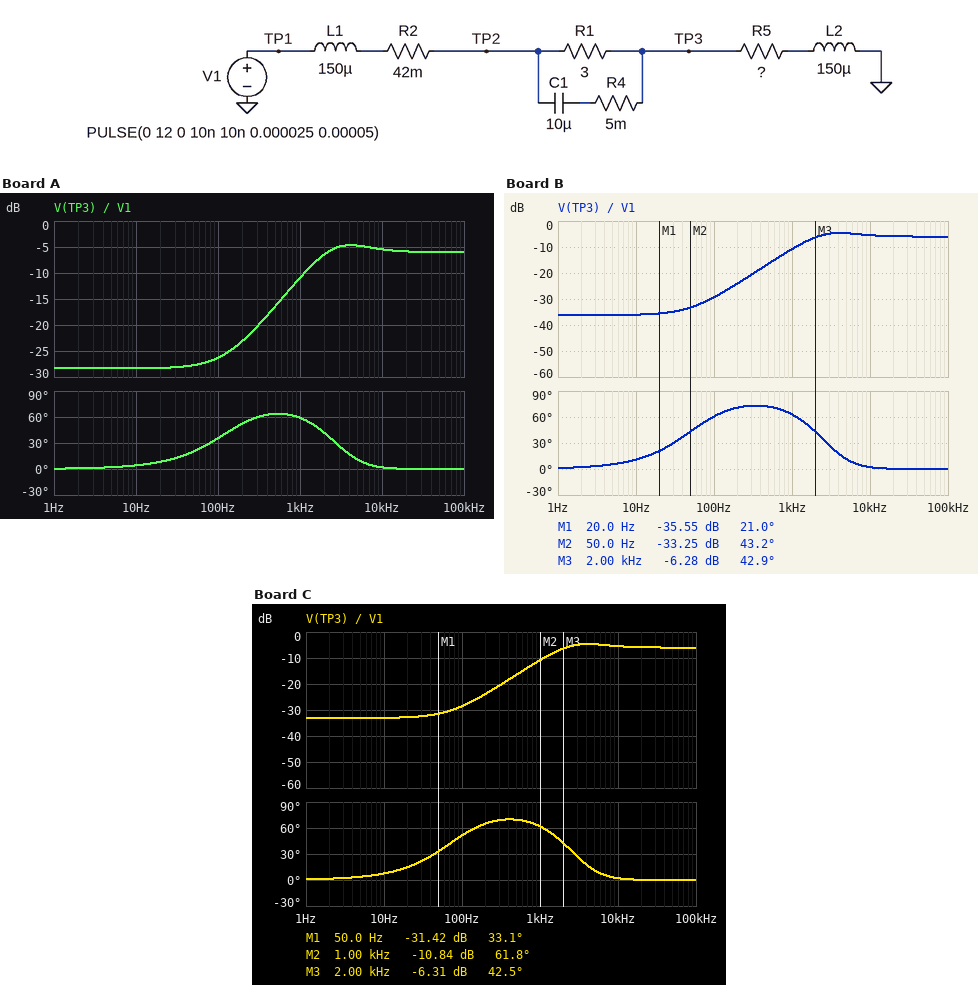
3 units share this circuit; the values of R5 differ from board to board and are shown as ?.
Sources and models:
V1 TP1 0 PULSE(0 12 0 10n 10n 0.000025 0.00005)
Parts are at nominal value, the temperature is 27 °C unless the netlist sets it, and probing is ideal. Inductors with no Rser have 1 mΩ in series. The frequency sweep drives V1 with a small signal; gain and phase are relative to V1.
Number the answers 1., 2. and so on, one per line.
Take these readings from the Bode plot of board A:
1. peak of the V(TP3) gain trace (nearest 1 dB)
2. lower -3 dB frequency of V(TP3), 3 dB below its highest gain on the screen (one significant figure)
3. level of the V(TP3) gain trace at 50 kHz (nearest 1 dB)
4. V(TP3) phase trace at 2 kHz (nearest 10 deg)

1. -5 dB
2. 2 kHz
3. -6 dB
4. 40 deg
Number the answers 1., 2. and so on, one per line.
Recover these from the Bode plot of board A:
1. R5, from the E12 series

1. 0.12 Ω
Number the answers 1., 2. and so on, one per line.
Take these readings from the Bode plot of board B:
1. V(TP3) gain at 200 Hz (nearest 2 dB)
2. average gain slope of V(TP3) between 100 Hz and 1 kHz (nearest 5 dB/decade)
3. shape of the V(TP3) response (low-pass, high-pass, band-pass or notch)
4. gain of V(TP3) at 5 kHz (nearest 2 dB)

1. -24 dB
2. 20 dB/decade
3. high-pass
4. -4 dB
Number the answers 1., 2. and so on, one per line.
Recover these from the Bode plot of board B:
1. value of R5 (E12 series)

1. 0.047 Ω
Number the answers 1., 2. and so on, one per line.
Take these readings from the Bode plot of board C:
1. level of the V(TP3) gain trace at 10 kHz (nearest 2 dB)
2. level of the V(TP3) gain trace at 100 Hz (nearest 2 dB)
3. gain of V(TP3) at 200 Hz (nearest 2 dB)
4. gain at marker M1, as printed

1. -6 dB
2. -28 dB
3. -24 dB
4. -31.42 dB
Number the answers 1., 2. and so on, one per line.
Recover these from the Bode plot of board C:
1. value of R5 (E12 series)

1. 0.068 Ω
